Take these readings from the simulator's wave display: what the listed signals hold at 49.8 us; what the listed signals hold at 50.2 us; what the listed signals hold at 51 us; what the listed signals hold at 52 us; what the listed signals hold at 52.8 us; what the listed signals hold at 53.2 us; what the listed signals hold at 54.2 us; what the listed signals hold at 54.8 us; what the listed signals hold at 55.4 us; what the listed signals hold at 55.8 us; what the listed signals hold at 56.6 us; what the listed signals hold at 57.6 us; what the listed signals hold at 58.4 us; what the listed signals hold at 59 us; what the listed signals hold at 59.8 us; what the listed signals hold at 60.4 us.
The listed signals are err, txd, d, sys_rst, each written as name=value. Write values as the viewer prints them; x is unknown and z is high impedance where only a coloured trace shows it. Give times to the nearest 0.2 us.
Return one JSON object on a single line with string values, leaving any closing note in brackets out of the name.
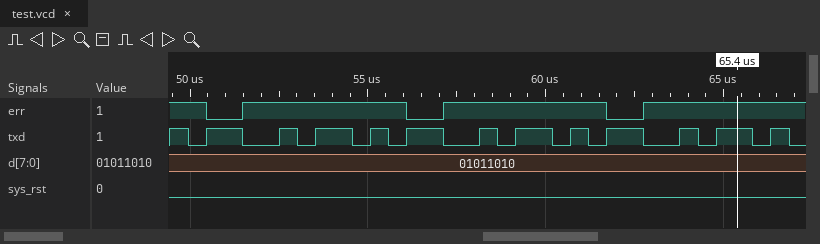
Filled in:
{"what the listed signals hold at 49.8 us": "err=1, txd=1, d=01011010, sys_rst=0", "what the listed signals hold at 50.2 us": "err=1, txd=0, d=01011010, sys_rst=0", "what the listed signals hold at 51 us": "err=0, txd=1, d=01011010, sys_rst=0", "what the listed signals hold at 52 us": "err=1, txd=0, d=01011010, sys_rst=0", "what the listed signals hold at 52.8 us": "err=1, txd=1, d=01011010, sys_rst=0", "what the listed signals hold at 53.2 us": "err=1, txd=0, d=01011010, sys_rst=0", "what the listed signals hold at 54.2 us": "err=1, txd=1, d=01011010, sys_rst=0", "what the listed signals hold at 54.8 us": "err=1, txd=0, d=01011010, sys_rst=0", "what the listed signals hold at 55.4 us": "err=1, txd=1, d=01011010, sys_rst=0", "what the listed signals hold at 55.8 us": "err=1, txd=0, d=01011010, sys_rst=0", "what the listed signals hold at 56.6 us": "err=0, txd=1, d=01011010, sys_rst=0", "what the listed signals hold at 57.6 us": "err=1, txd=0, d=01011010, sys_rst=0", "what the listed signals hold at 58.4 us": "err=1, txd=1, d=01011010, sys_rst=0", "what the listed signals hold at 59 us": "err=1, txd=0, d=01011010, sys_rst=0", "what the listed signals hold at 59.8 us": "err=1, txd=1, d=01011010, sys_rst=0", "what the listed signals hold at 60.4 us": "err=1, txd=0, d=01011010, sys_rst=0"}
